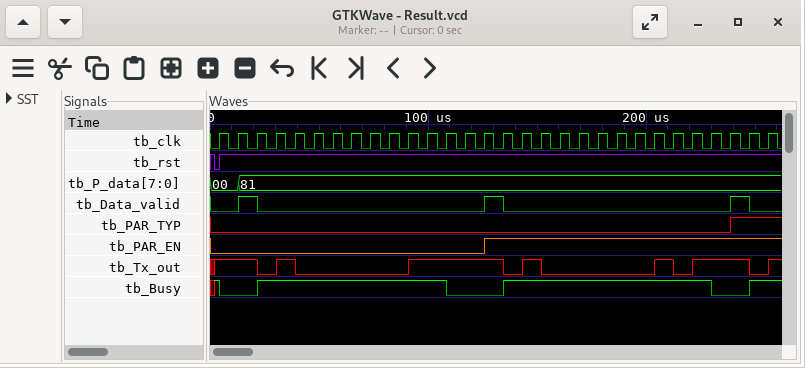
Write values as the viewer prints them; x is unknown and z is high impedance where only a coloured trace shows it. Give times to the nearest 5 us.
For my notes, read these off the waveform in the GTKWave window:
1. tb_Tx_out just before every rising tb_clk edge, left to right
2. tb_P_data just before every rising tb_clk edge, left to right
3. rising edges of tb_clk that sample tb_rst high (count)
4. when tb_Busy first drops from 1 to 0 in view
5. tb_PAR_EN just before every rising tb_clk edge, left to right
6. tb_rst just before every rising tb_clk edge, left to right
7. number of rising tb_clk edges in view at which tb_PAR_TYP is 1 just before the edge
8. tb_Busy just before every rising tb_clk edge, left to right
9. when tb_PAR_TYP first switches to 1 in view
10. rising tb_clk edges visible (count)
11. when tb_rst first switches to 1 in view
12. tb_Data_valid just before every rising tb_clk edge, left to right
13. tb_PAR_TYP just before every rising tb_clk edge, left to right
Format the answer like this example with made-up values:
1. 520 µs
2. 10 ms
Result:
1. 1 1 1 0 1 0 0 0 0 0 0 1 1 1 1 1 0 1 0 0 0 0 0 0 1 0 1 1 1 0
2. 00, 00, 81, 81, 81, 81, 81, 81, 81, 81, 81, 81, 81, 81, 81, 81, 81, 81, 81, 81, 81, 81, 81, 81, 81, 81, 81, 81, 81, 81
3. 29
4. 5 us
5. 0 0 0 0 0 0 0 0 0 0 0 0 0 0 0 1 1 1 1 1 1 1 1 1 1 1 1 1 1 1
6. 0 1 1 1 1 1 1 1 1 1 1 1 1 1 1 1 1 1 1 1 1 1 1 1 1 1 1 1 1 1
7. 2
8. 1 0 0 1 1 1 1 1 1 1 1 1 1 0 0 0 1 1 1 1 1 1 1 1 1 1 1 0 0 1
9. 240 us
10. 30
11. 5 us
12. 0 0 1 0 0 0 0 0 0 0 0 0 0 0 0 1 0 0 0 0 0 0 0 0 0 0 0 0 1 0
13. 0 0 0 0 0 0 0 0 0 0 0 0 0 0 0 0 0 0 0 0 0 0 0 0 0 0 0 0 1 1
